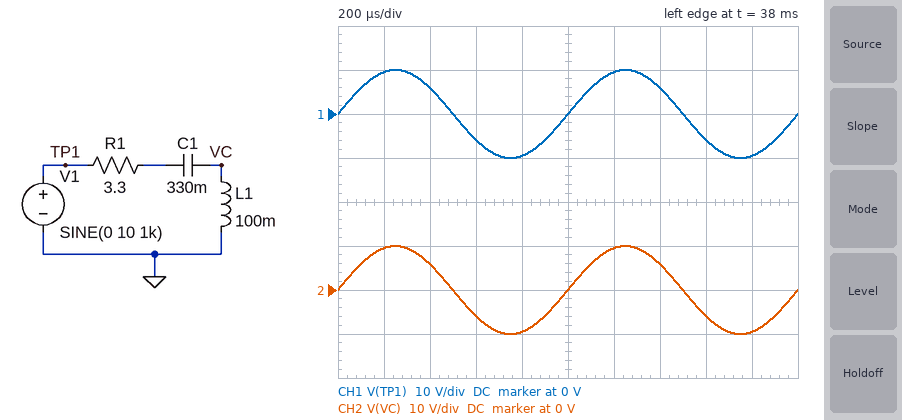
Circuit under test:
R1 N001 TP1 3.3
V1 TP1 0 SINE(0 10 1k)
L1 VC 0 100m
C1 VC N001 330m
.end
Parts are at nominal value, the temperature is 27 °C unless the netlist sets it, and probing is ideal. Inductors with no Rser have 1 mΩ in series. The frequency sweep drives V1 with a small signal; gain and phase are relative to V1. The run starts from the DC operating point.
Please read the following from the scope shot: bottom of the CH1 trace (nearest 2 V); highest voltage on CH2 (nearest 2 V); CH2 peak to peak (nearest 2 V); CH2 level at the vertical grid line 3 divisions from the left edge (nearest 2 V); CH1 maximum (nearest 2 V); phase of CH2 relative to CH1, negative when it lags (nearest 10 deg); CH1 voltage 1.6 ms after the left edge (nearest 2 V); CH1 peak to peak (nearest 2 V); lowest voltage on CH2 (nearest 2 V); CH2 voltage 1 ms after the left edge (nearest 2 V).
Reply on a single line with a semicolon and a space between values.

-10 V; 10 V; 20 V; -6 V; 10 V; 0 deg; -6 V; 20 V; -10 V; 0 V
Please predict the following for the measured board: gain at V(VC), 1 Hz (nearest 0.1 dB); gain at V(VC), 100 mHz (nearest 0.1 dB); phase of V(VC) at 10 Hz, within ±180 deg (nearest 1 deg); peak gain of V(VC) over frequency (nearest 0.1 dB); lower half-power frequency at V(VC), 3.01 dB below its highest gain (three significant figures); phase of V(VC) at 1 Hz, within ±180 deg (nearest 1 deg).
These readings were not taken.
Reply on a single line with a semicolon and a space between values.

-14.4 dB; -39.3 dB; 28 deg; 0 dB; 5.11 Hz; 87 deg
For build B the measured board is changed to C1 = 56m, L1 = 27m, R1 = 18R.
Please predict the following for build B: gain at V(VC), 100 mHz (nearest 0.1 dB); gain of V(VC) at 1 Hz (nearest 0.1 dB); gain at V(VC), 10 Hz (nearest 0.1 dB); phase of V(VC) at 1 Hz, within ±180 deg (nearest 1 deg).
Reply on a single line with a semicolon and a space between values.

-65.9 dB; -40.6 dB; -20.5 dB; 98 deg
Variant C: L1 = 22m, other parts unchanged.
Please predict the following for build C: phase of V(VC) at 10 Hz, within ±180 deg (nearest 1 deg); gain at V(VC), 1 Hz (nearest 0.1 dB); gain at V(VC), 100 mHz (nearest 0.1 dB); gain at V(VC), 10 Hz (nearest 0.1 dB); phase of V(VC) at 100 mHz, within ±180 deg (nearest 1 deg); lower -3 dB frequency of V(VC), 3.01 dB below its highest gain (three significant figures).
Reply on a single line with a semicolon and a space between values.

68 deg; -27.6 dB; -52.5 dB; -8.2 dB; 141 deg; 23.7 Hz
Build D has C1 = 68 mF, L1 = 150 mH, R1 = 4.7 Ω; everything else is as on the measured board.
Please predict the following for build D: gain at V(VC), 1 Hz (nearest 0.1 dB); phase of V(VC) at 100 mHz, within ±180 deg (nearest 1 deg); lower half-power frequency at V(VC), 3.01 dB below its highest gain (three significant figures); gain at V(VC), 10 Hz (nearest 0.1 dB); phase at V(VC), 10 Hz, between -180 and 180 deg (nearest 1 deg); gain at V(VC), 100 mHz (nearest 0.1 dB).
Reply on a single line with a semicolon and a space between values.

-14.3 dB; 168 deg; 4.50 Hz; -0.8 dB; 27 deg; -48.0 dB
